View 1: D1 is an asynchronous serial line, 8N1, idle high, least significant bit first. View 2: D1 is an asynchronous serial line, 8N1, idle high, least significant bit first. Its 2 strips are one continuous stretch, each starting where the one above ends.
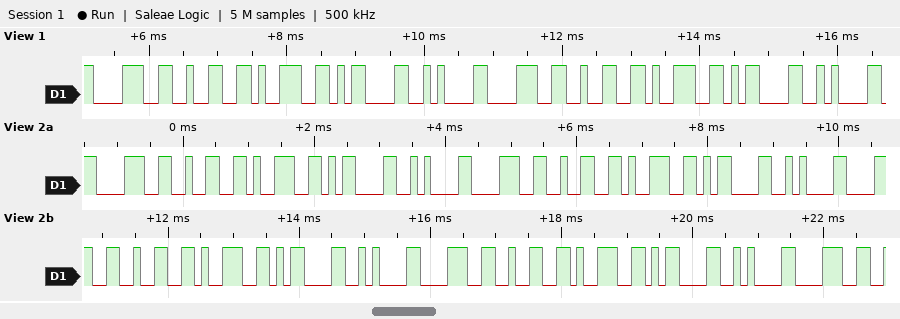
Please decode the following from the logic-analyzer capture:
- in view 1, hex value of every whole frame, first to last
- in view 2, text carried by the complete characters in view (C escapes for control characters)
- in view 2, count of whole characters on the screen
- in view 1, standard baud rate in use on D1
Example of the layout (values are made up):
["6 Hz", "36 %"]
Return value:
["0x38 0x32 0x39 0x0D 0x0A 0x38 0x32 0x39 0x0D 0x0A", "\"829\\r\\n829\\r\\n829\\r\\n829\\r\\n8\"", "21", "9600 baud"]
